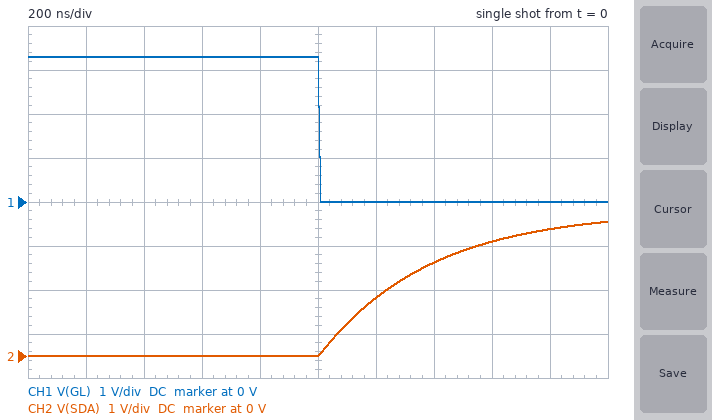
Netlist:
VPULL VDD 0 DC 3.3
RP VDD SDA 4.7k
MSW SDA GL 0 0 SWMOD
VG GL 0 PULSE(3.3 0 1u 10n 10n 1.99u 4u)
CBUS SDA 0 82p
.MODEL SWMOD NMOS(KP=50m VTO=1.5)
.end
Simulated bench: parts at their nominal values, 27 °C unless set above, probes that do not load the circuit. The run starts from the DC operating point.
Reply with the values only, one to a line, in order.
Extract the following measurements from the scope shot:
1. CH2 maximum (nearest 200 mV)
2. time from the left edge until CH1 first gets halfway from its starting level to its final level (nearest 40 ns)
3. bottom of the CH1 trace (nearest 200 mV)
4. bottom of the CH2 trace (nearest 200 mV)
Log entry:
3.0 V
1.00 µs
0 V
0 V
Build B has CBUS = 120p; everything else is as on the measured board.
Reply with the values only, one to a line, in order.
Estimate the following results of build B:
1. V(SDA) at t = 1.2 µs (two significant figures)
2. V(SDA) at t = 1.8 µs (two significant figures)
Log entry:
980 mV
2.5 V
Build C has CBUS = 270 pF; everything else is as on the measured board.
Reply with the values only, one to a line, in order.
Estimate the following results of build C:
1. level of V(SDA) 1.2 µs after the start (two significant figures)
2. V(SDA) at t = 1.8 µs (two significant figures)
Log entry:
480 mV
1.5 V
